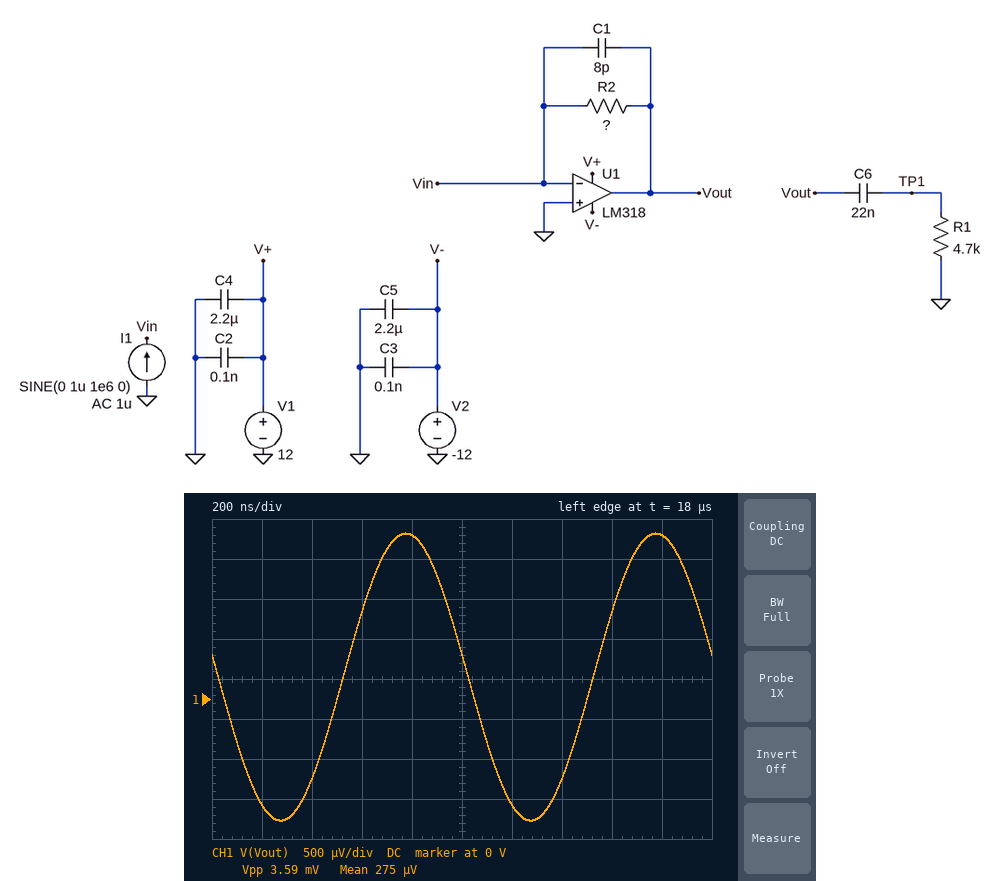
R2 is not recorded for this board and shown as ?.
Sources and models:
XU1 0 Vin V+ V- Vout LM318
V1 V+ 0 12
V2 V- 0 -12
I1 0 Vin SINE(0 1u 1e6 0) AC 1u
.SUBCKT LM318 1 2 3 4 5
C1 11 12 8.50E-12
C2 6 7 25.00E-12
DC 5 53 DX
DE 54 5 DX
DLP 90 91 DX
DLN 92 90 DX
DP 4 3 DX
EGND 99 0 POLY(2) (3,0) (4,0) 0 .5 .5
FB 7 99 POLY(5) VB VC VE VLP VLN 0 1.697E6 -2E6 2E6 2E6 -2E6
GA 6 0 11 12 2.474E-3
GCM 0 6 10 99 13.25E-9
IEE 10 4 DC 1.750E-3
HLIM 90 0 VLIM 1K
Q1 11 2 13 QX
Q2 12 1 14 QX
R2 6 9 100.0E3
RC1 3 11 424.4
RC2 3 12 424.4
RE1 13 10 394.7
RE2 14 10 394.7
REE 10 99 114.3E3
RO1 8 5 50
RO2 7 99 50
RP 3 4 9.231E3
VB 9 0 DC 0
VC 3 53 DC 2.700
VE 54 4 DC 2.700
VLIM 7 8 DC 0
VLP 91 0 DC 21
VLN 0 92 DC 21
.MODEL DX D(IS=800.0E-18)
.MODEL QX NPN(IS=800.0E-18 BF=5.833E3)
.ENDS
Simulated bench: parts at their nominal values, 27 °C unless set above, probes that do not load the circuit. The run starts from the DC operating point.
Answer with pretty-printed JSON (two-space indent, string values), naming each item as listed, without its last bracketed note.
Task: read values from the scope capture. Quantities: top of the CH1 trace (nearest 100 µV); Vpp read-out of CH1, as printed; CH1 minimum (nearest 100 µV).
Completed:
{
  "top of the CH1 trace": "2.1 mV",
  "Vpp read-out of CH1, as printed": "3.59 mV",
  "CH1 minimum": "-1.5 mV"
}
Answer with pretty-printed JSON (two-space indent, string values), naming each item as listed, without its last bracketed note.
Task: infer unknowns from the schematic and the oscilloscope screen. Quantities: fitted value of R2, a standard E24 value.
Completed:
{
  "fitted value of R2, a standard E24 value": "1.8 kΩ"
}
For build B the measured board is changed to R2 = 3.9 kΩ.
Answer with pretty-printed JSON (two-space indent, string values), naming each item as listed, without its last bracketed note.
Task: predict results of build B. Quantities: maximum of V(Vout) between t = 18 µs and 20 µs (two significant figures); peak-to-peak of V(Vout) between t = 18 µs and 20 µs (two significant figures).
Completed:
{
  "maximum of V(Vout) between t = 18 µs and 20 µs": "4.4 mV",
  "peak-to-peak of V(Vout) between t = 18 µs and 20 µs": "7.7 mV"
}
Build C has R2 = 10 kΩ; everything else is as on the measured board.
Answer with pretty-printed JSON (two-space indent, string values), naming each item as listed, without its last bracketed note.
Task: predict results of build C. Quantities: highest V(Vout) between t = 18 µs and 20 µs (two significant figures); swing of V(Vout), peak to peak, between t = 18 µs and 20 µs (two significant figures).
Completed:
{
  "highest V(Vout) between t = 18 µs and 20 µs": "10 mV",
  "swing of V(Vout), peak to peak, between t = 18 µs and 20 µs": "18 mV"
}
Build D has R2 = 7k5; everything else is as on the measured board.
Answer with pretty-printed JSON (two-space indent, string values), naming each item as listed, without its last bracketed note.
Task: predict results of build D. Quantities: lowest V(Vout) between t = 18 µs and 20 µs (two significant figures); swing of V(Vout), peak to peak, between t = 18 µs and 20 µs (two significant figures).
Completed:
{
  "lowest V(Vout) between t = 18 µs and 20 µs": "-5.9 mV",
  "swing of V(Vout), peak to peak, between t = 18 µs and 20 µs": "14 mV"
}
